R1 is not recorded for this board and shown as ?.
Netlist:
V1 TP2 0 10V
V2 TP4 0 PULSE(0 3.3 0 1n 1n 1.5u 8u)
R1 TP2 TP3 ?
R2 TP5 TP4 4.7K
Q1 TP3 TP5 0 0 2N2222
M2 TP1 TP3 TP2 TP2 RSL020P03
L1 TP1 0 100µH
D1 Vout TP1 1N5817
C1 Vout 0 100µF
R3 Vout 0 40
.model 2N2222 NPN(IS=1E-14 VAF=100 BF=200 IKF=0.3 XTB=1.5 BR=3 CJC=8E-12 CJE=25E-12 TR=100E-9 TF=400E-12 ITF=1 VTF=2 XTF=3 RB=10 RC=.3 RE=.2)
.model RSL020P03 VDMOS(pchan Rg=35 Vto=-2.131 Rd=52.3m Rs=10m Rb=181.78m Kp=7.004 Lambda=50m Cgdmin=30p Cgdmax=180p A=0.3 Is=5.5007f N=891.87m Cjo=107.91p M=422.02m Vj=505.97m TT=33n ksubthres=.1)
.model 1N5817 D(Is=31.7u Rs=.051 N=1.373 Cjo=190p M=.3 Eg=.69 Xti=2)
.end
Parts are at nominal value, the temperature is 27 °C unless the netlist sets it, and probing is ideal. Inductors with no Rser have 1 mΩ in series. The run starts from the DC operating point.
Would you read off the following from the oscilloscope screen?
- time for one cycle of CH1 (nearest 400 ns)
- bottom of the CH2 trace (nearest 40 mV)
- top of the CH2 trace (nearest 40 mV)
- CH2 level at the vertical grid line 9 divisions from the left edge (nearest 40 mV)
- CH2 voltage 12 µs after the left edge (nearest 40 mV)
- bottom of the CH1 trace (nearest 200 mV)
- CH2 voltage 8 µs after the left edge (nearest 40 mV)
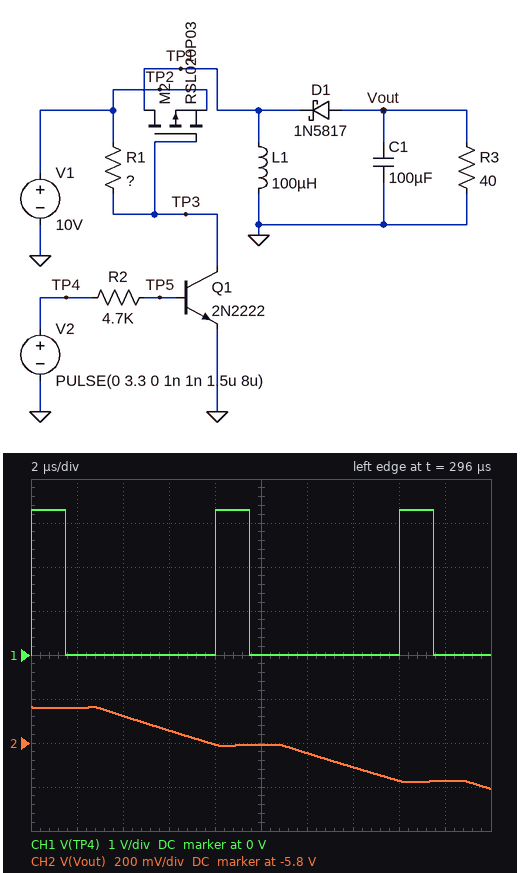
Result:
8.0 µs
-6.00 V
-5.64 V
-5.96 V
-5.84 V
0 V
-5.80 V
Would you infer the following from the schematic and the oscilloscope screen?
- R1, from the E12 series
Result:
390 Ω
